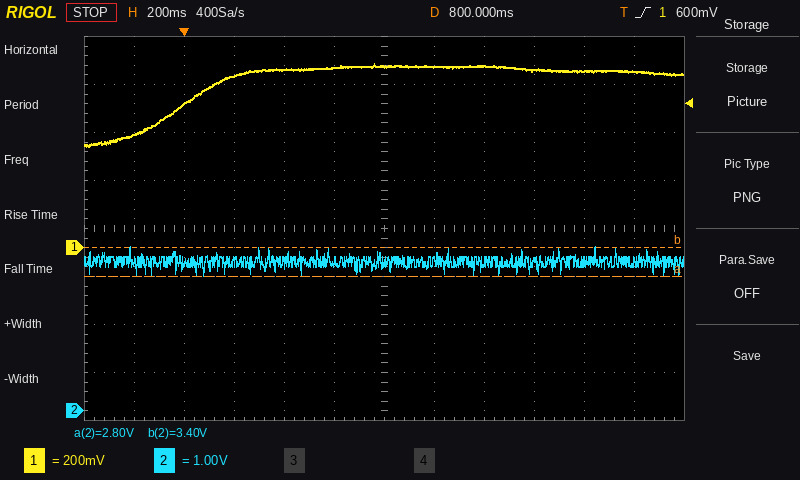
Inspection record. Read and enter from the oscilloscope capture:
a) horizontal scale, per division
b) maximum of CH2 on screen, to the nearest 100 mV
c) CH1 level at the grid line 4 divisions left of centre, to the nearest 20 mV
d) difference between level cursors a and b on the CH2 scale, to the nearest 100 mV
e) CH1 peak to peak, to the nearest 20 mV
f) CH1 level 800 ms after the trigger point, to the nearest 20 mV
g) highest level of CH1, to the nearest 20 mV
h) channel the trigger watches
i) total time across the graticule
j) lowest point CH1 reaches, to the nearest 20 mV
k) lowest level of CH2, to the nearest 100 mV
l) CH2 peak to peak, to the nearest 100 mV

200 ms
3.4 V
600 mV
600 mV
340 mV
760 mV
760 mV
CH1
2.4 s
420 mV
2.8 V
600 mV
